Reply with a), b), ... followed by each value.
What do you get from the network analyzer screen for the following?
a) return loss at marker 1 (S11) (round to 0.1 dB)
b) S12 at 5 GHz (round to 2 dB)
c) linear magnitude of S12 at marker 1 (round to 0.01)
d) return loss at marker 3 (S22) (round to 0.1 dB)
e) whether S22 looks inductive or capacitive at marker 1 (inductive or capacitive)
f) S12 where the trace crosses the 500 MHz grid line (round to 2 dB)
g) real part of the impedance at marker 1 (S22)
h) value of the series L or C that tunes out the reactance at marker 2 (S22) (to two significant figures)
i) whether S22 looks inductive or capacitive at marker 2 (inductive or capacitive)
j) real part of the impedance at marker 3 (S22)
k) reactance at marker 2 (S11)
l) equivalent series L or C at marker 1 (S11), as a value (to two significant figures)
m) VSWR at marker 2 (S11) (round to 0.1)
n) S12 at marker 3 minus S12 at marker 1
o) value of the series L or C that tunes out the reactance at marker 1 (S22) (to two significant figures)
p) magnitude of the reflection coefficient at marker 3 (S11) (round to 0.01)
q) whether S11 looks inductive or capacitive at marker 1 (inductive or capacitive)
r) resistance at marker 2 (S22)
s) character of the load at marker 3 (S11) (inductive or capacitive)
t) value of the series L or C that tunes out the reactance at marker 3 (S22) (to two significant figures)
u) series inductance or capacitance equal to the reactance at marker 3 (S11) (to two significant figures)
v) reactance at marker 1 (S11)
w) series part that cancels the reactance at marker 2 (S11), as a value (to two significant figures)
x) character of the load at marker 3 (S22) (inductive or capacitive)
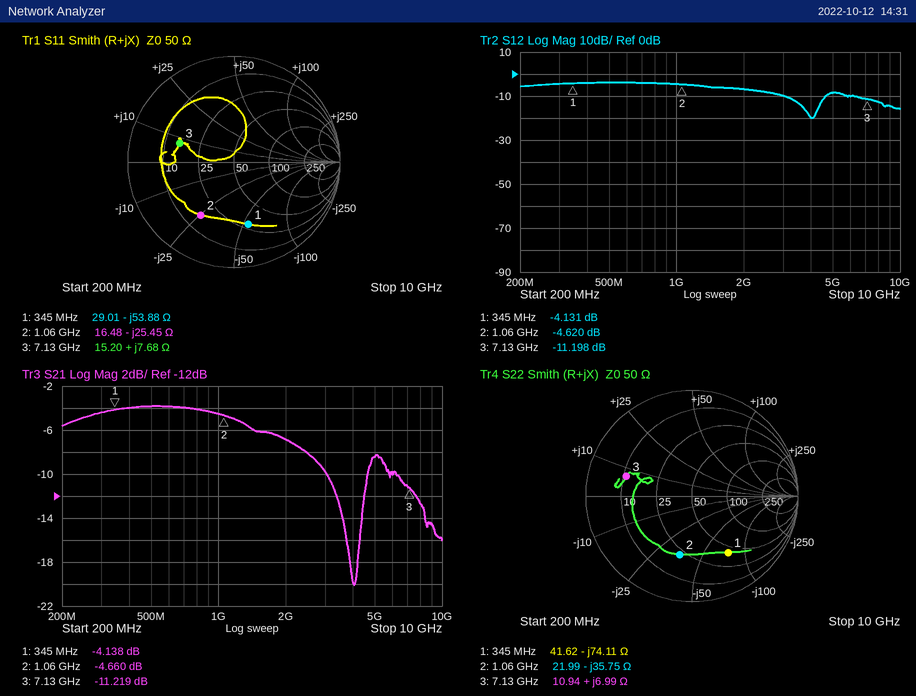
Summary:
a) 4.4 dB
b) -8 dB
c) 0.62
d) 3.8 dB
e) capacitive
f) -4 dB
g) 41.62 Ω
h) 5.4 nH
i) capacitive
j) 10.94 Ω
k) -25.45 Ω
l) 8.6 pF
m) 3.9
n) -7.067 dB
o) 34 nH
p) 0.54
q) capacitive
r) 21.99 Ω
s) inductive
t) 3.2 pF
u) 170 pH
v) -53.88 Ω
w) 3.8 nH
x) inductive
